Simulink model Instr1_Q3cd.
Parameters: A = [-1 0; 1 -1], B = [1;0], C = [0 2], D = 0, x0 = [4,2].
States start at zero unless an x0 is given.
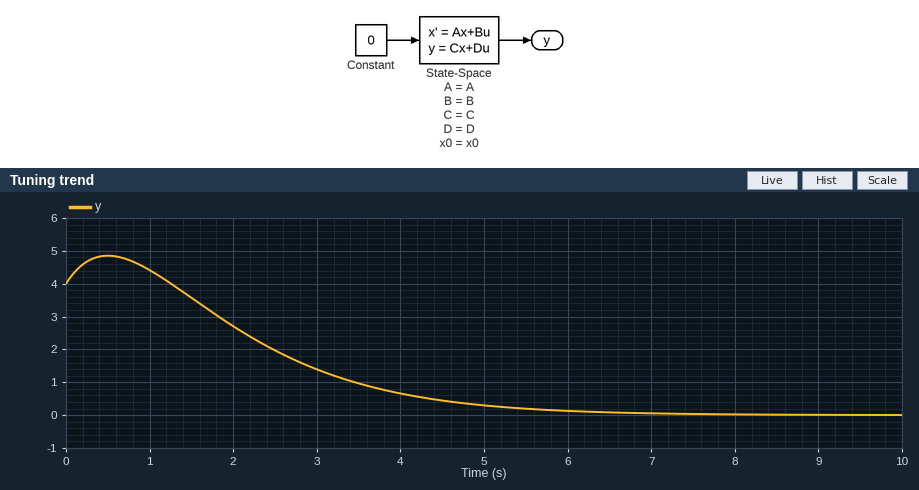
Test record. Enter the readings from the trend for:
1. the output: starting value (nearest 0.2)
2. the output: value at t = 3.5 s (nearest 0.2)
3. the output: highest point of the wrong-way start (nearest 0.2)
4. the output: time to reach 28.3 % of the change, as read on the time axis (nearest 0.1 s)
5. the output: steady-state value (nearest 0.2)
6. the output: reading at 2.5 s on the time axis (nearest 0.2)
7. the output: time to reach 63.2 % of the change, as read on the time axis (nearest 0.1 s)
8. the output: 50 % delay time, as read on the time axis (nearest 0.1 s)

4.0
1.0
4.8
1.9 s
0.0
2.0
2.9 s
2.5 s
